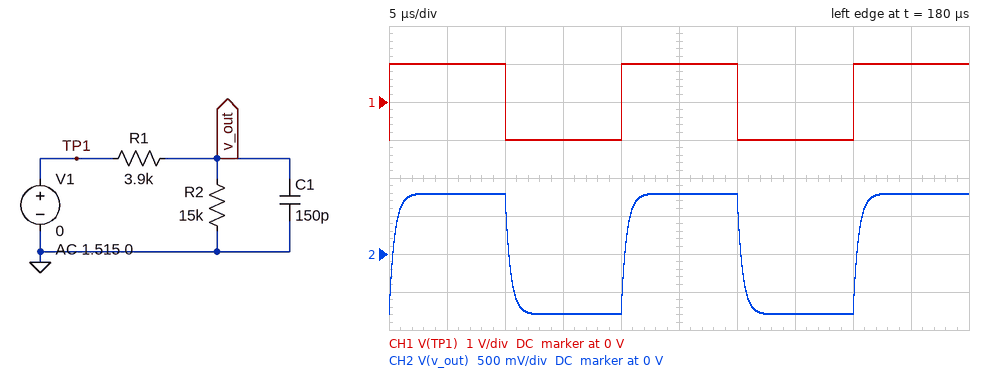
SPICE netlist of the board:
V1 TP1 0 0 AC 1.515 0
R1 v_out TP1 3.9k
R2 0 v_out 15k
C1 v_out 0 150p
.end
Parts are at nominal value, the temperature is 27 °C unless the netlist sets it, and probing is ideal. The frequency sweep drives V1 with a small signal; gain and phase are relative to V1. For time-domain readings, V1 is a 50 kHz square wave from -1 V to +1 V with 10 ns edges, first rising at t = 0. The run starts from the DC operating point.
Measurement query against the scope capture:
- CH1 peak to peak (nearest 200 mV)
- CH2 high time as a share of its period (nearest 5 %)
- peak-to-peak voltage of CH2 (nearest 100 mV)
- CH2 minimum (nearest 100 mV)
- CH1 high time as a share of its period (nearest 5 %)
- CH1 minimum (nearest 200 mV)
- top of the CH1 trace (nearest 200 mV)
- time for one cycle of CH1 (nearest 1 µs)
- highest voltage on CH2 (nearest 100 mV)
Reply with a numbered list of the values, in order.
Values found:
1. 2.0 V
2. 50 %
3. 1.6 V
4. -800 mV
5. 50 %
6. -1.0 V
7. 1.0 V
8. 20 µs
9. 800 mV
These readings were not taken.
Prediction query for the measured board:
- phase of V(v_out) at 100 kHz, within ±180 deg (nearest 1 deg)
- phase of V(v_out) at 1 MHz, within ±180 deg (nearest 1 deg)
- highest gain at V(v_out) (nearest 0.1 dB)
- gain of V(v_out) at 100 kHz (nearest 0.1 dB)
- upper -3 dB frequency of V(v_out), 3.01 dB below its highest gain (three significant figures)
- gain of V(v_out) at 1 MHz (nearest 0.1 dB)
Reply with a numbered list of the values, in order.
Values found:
1. -16 deg
2. -71 deg
3. -2.0 dB
4. -2.4 dB
5. 343 kHz
6. -11.8 dB
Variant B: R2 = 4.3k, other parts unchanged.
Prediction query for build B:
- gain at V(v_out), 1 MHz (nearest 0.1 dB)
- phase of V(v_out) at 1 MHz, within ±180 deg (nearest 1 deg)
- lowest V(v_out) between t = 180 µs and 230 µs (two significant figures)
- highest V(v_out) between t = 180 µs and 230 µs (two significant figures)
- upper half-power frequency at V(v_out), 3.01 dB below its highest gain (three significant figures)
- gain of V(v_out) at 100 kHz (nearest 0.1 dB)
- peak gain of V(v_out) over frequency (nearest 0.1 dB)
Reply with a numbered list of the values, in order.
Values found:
1. -12.3 dB
2. -63 deg
3. -520 mV
4. 520 mV
5. 519 kHz
6. -5.8 dB
7. -5.6 dB
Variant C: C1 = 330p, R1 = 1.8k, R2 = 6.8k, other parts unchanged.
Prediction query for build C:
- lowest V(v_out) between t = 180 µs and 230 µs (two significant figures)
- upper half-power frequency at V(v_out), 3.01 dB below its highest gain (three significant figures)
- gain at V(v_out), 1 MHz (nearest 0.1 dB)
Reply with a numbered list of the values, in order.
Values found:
1. -790 mV
2. 339 kHz
3. -11.9 dB
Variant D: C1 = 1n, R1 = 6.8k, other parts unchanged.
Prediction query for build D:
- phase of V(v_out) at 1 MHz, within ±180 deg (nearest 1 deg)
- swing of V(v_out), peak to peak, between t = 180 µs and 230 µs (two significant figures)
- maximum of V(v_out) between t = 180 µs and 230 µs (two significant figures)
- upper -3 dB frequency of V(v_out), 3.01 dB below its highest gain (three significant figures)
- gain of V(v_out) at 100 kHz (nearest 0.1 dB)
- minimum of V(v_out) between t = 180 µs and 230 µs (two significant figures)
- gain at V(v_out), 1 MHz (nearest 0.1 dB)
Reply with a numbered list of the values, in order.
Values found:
1. -88 deg
2. 1.1 V
3. 540 mV
4. 34.0 kHz
5. -13.1 dB
6. -540 mV
7. -32.6 dB
